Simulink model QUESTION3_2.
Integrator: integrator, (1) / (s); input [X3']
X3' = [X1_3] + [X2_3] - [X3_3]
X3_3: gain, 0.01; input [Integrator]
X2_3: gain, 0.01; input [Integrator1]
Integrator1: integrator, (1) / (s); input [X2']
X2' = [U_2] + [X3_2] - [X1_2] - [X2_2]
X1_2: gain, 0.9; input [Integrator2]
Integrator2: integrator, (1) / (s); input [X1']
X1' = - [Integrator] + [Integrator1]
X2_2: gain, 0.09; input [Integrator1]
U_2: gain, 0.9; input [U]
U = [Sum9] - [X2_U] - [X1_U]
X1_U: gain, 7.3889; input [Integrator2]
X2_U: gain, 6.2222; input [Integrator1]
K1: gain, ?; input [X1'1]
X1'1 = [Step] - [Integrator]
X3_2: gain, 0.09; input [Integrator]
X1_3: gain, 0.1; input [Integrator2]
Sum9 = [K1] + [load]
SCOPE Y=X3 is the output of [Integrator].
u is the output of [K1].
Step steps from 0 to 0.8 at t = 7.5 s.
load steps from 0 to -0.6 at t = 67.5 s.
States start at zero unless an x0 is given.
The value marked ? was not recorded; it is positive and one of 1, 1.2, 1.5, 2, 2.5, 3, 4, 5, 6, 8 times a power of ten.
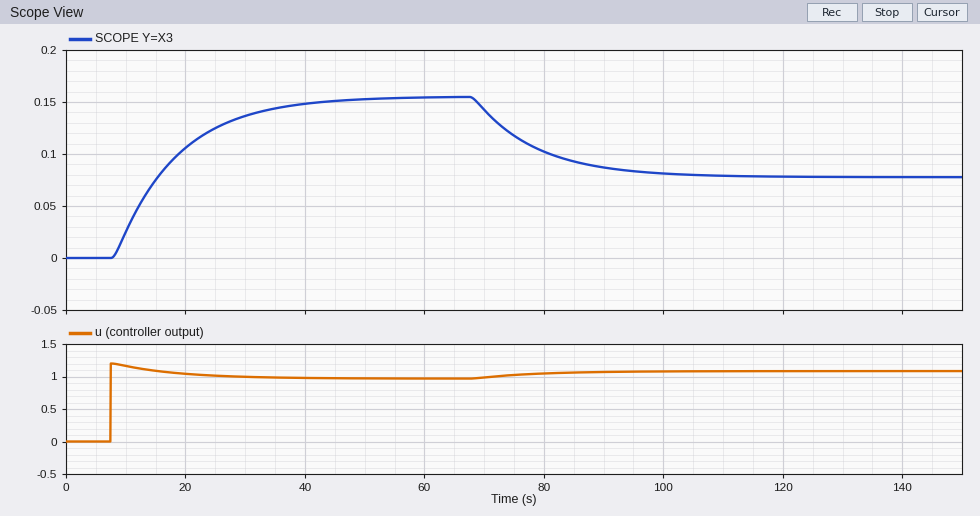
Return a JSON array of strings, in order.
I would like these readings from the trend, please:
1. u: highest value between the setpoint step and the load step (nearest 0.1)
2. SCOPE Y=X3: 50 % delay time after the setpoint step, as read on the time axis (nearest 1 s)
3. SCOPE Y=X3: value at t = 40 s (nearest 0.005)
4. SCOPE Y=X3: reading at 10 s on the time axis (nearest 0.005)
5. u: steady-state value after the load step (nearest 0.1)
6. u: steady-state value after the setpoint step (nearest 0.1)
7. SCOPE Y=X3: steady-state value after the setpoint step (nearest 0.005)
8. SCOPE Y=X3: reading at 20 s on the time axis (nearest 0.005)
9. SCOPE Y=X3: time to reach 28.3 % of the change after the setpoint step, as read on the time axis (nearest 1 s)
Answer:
["1.2", "15 s", "0.150", "0.025", "1.1", "1.0", "0.155", "0.105", "12 s"]
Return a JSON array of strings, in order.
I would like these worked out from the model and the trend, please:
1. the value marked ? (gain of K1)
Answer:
["1.5"]
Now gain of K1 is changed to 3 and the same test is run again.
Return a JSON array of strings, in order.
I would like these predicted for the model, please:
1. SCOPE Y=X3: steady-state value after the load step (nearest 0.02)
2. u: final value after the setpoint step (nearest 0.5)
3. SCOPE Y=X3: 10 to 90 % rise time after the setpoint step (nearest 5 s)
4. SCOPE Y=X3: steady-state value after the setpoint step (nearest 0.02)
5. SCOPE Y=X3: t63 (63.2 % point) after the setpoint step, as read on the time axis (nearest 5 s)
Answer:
["0.20", "1.5", "20 s", "0.26", "15 s"]
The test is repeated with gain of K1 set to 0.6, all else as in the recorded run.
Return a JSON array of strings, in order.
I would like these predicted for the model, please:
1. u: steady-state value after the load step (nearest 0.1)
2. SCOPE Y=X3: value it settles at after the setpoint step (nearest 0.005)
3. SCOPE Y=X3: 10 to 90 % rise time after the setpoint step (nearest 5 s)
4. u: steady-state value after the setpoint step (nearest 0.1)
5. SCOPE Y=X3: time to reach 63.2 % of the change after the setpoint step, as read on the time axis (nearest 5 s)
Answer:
["0.5", "0.070", "25 s", "0.4", "20 s"]
